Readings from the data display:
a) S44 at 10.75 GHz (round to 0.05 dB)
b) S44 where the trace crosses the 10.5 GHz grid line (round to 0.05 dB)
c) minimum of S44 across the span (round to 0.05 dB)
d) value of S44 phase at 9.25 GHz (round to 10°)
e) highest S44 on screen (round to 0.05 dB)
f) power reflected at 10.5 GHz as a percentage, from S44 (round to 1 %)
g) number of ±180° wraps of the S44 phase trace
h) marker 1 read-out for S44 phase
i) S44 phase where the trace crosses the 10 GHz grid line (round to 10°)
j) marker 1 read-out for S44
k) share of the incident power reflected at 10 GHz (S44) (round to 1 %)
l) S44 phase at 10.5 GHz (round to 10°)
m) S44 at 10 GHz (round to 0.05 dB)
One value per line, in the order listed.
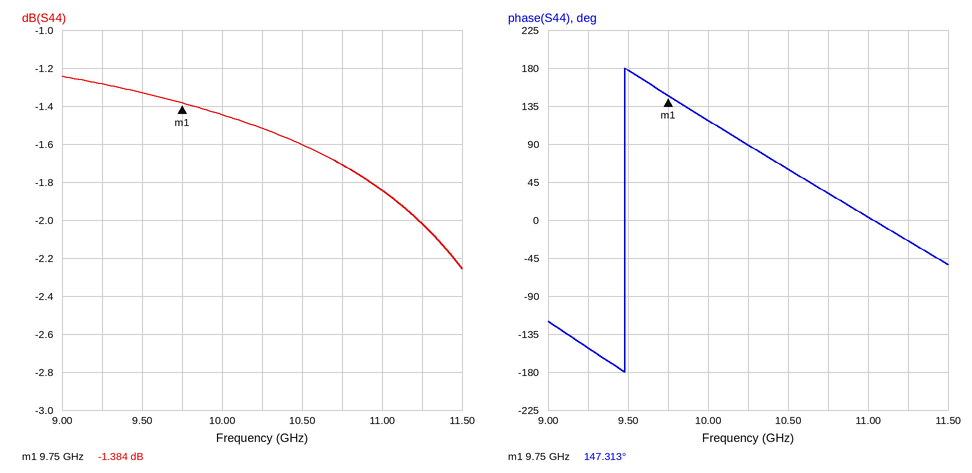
-1.70 dB
-1.60 dB
-2.25 dB
-150°
-1.25 dB
69 %
1
147.313°
120°
-1.384 dB
72 %
60°
-1.45 dB
